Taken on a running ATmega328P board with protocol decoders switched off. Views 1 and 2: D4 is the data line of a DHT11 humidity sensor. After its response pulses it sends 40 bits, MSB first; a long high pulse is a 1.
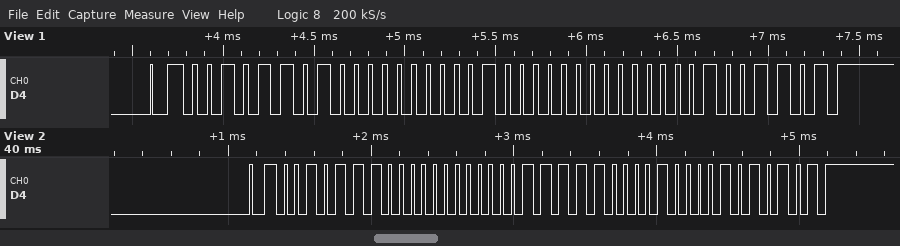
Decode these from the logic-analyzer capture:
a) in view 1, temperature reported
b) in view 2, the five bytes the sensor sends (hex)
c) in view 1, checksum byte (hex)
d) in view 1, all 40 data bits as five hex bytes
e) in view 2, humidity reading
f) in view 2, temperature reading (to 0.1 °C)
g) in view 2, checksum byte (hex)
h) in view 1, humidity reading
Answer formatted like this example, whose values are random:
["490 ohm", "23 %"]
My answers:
["32.0 °C", "2E 00 1F 08 55", "0x4D", "2D 00 20 00 4D", "46 %", "31.8 °C", "0x55", "45 %"]
